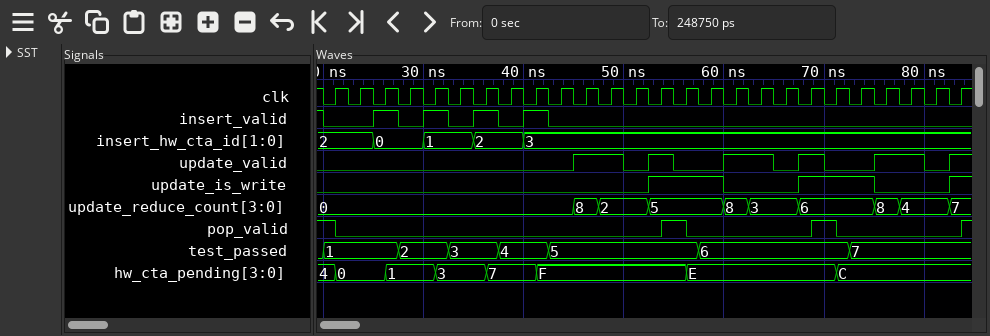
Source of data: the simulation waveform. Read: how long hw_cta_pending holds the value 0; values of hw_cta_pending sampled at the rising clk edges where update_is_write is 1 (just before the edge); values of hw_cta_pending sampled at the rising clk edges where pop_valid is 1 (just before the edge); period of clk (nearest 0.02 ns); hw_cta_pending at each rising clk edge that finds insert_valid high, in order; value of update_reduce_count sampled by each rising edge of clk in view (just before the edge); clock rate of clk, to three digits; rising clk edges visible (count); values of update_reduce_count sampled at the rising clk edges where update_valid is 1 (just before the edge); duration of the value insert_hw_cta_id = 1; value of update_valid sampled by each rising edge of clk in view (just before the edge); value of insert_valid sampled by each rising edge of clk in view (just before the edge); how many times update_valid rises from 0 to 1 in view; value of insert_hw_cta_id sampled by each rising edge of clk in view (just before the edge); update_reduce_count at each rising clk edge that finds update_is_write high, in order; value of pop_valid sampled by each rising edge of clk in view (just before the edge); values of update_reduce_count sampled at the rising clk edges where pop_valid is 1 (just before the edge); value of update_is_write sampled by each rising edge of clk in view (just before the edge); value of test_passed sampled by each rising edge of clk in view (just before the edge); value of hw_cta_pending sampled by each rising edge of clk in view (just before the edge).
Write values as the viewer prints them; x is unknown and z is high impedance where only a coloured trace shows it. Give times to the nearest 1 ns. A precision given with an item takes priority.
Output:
5 ns
F, F, E, E, E, C, C
4, F, E
2.5 ns
0, 1, 3, 7
0, 0, 0, 0, 0, 0, 0, 0, 0, 0, 8, 2, 2, 5, 5, 5, 8, 3, 3, 6, 6, 6, 8, 4, 4, 7
400 MHz
26
8, 2, 5, 8, 3, 6, 8, 4, 7
5 ns
0 0 0 0 0 0 0 0 0 0 1 1 0 1 0 0 1 1 0 1 0 0 1 1 0 1
0 0 1 0 1 0 1 0 1 0 0 0 0 0 0 0 0 0 0 0 0 0 0 0 0 0
6
2, 2, 0, 0, 1, 1, 2, 2, 3, 3, 3, 3, 3, 3, 3, 3, 3, 3, 3, 3, 3, 3, 3, 3, 3, 3
5, 5, 5, 6, 6, 6, 7
1 0 0 0 0 0 0 0 0 0 0 0 0 0 1 0 0 0 0 0 1 0 0 0 0 0
0, 5, 6
0 0 0 0 0 0 0 0 0 0 0 0 0 1 1 1 0 0 0 1 1 1 0 0 0 1
1, 1, 1, 2, 2, 3, 3, 4, 4, 5, 5, 5, 5, 5, 5, 6, 6, 6, 6, 6, 6, 7, 7, 7, 7, 7
4, 0, 0, 1, 1, 3, 3, 7, 7, F, F, F, F, F, F, E, E, E, E, E, E, C, C, C, C, C
